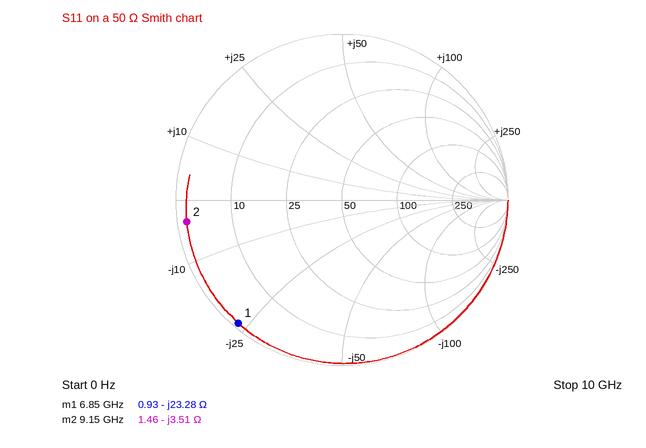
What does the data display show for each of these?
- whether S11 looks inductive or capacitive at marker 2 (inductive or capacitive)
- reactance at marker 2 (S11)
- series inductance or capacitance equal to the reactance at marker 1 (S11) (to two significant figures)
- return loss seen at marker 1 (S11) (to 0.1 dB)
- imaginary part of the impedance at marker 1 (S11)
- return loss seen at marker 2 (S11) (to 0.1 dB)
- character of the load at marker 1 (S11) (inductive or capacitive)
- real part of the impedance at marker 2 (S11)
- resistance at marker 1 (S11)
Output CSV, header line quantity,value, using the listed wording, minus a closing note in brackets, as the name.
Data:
quantity,value
whether S11 looks inductive or capacitive at marker 2,capacitive
reactance at marker 2,-3.51 Ω
series inductance or capacitance equal to the reactance at marker 1 (S11),1.00 pF
return loss seen at marker 1 (S11),0.3 dB
imaginary part of the impedance at marker 1,-23.28 Ω
return loss seen at marker 2 (S11),0.5 dB
character of the load at marker 1 (S11),capacitive
real part of the impedance at marker 2,1.46 Ω
resistance at marker 1,0.93 Ω
